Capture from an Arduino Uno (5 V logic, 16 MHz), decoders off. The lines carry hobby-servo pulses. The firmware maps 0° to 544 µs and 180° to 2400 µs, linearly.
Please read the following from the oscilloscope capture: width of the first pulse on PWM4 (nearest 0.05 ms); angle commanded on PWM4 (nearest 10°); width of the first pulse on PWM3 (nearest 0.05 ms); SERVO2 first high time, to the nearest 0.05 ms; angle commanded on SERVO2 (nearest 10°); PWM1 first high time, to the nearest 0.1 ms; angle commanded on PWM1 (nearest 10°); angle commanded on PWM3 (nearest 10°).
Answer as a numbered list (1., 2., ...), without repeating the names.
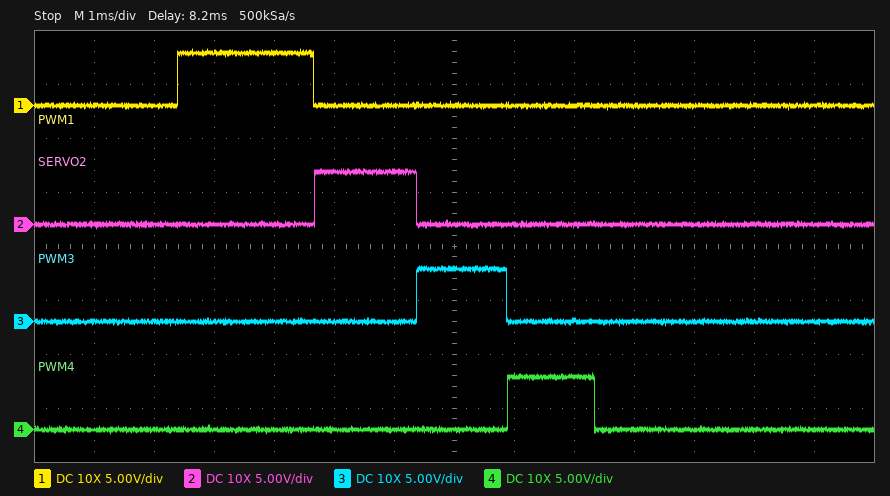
1. 1.45 ms
2. 90°
3. 1.50 ms
4. 1.70 ms
5. 110°
6. 2.3 ms
7. 170°
8. 90°
